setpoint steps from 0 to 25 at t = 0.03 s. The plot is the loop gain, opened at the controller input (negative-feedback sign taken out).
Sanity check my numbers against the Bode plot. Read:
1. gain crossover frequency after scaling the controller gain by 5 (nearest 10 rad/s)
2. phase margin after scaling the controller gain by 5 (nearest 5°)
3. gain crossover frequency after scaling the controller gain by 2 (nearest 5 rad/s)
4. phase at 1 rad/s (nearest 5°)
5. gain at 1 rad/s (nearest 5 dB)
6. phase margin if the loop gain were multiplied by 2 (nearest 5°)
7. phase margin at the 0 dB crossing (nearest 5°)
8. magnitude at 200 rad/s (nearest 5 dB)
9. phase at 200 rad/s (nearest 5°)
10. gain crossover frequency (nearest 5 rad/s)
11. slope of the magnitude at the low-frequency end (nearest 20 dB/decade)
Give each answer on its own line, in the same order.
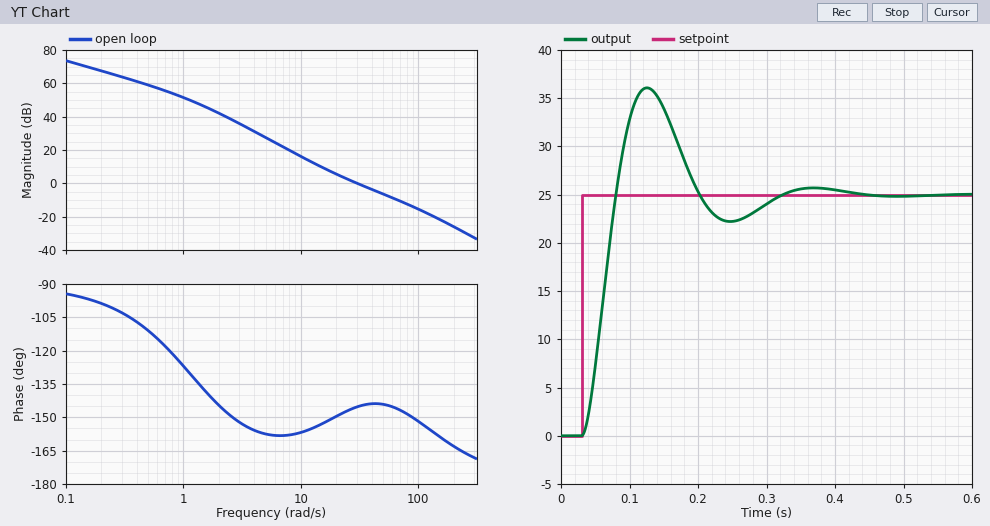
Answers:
90 rad/s
30°
50 rad/s
-125°
50 dB
35°
35°
-25 dB
-165°
30 rad/s
-20 dB/decade
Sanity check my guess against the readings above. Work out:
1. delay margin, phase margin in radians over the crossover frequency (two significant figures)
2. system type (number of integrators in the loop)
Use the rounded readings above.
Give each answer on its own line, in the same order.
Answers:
0.020 s
1
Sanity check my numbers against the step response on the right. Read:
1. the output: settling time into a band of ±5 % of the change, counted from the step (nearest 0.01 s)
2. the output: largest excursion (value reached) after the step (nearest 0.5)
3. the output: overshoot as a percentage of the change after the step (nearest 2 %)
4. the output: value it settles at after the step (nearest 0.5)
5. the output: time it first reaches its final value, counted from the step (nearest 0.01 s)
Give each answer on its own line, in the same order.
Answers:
0.26 s
36.0
44 %
25.0
0.05 s
